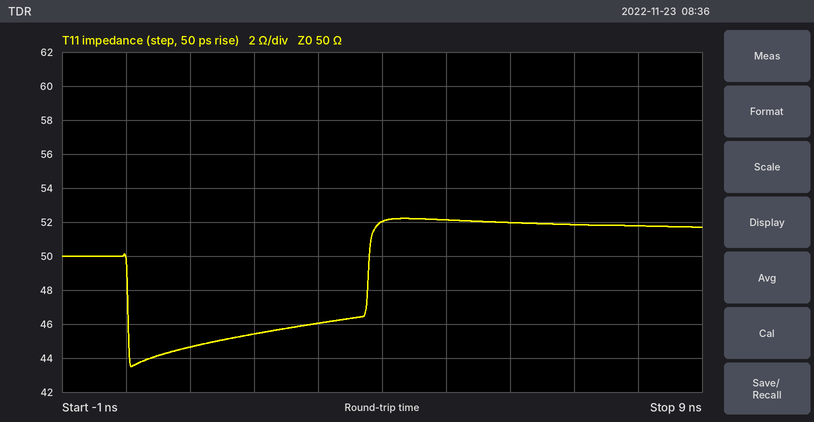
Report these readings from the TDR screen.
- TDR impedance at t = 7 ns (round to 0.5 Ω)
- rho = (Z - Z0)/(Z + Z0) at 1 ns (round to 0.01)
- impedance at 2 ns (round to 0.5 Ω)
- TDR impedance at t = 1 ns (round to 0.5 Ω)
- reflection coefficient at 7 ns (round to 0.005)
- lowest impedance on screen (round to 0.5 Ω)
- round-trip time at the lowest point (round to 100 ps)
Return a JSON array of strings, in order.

["52.0 Ω", "-0.06", "45.5 Ω", "44.5 Ω", "+0.020", "43.5 Ω", "100 ps"]
